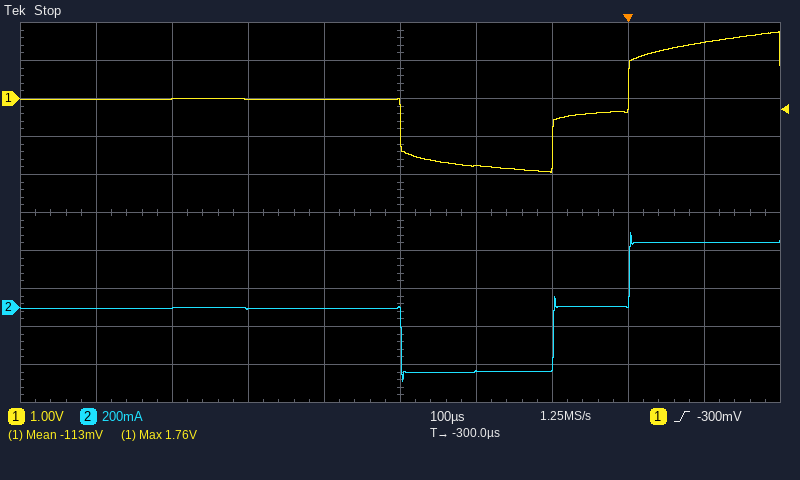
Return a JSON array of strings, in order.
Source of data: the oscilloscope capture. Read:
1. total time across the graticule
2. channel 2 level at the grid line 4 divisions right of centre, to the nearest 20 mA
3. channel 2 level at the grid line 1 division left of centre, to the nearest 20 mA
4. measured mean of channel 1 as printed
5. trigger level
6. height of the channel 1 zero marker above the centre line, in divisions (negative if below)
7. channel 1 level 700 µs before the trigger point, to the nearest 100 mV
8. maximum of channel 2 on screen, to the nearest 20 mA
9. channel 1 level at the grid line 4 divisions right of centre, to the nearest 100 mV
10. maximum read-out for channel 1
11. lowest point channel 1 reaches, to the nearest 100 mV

["1 ms", "340 mA", "0 mA", "-113 mV", "-300 mV", "+3.0 div", "0.0 V", "400 mA", "1.5 V", "1.76 V", "-1.9 V"]
